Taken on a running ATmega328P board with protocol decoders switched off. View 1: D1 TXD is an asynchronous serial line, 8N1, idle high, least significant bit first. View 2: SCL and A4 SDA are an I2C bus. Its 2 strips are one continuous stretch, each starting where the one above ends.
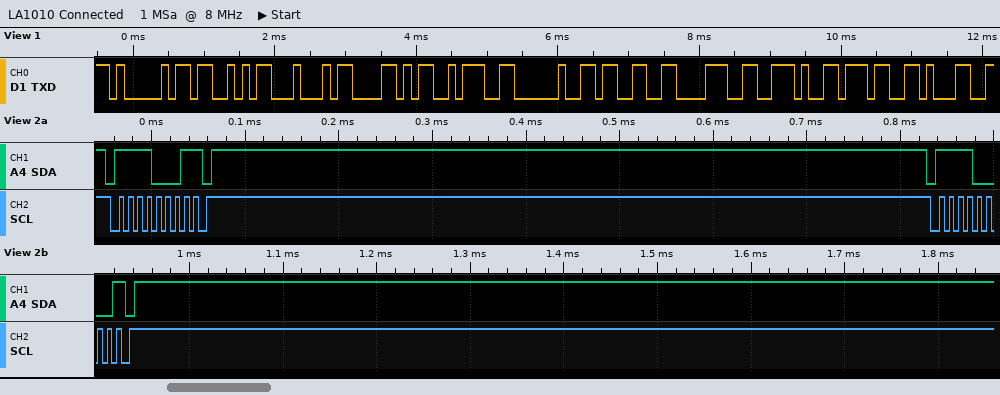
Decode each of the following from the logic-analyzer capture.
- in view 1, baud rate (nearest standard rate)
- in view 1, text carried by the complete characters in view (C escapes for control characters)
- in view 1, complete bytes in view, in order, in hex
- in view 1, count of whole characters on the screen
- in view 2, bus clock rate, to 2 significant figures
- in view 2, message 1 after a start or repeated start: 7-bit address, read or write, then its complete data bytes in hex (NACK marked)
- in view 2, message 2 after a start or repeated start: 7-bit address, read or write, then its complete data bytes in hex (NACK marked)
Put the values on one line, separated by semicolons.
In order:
9600 baud; "ASDX: 38.71"; 41 53 44 58 3A 20 33 38 2E 37 31; 11; 100 kHz; 0x78 read NACK; 0x78 write NACK
